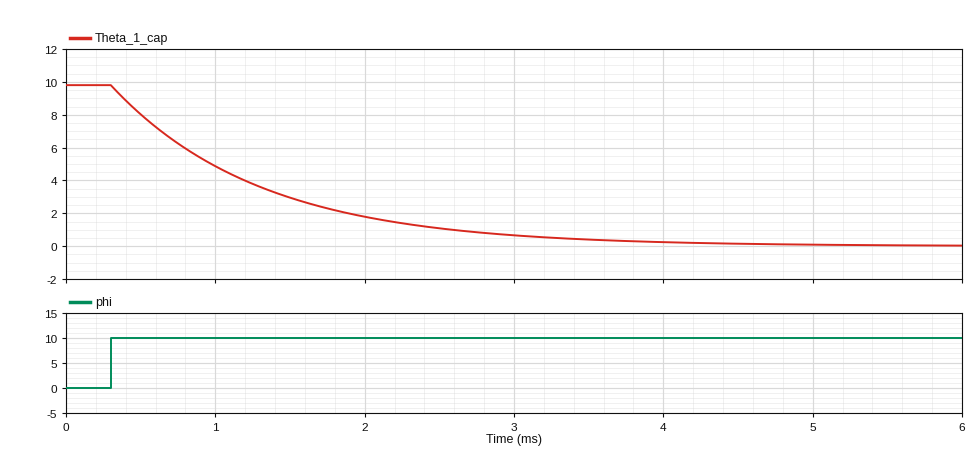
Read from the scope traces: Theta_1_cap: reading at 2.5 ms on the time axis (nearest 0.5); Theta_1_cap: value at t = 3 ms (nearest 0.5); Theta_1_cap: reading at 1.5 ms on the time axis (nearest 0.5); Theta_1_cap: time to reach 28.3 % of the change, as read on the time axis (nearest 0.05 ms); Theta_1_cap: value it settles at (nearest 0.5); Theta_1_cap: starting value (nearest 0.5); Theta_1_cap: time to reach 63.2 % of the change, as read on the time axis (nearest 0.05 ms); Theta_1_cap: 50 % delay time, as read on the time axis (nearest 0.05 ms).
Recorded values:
1.0
0.5
3.0
0.65 ms
0.0
10.0
1.30 ms
1.00 ms
